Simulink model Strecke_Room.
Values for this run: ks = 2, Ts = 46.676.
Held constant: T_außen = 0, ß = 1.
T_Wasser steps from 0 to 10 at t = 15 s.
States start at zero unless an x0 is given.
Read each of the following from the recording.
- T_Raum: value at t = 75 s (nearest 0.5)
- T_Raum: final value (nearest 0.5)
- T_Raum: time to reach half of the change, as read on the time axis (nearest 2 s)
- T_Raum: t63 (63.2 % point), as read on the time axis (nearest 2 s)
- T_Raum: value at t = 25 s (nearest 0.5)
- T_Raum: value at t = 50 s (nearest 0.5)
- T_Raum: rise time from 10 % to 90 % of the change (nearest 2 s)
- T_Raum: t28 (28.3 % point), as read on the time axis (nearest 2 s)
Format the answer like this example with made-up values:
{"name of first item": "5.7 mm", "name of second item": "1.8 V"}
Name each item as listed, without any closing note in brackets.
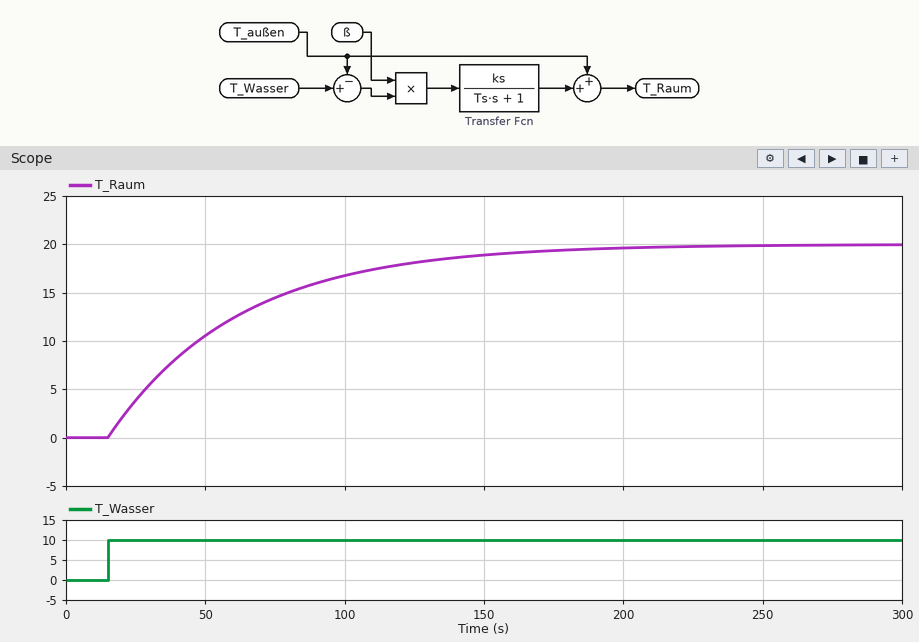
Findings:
{"T_Raum: value at t = 75 s": "14.5", "T_Raum: final value": "20.0", "T_Raum: time to reach half of the change, as read on the time axis": "48 s", "T_Raum: t63 (63.2 % point), as read on the time axis": "62 s", "T_Raum: value at t = 25 s": "4.0", "T_Raum: value at t = 50 s": "10.5", "T_Raum: rise time from 10 % to 90 % of the change": "102 s", "T_Raum: t28 (28.3 % point), as read on the time axis": "30 s"}
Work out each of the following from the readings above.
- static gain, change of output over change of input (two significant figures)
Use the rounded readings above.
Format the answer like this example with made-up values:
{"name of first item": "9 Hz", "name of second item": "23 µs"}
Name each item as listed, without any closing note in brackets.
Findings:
{"static gain, change of output over change of input": "2.0"}
